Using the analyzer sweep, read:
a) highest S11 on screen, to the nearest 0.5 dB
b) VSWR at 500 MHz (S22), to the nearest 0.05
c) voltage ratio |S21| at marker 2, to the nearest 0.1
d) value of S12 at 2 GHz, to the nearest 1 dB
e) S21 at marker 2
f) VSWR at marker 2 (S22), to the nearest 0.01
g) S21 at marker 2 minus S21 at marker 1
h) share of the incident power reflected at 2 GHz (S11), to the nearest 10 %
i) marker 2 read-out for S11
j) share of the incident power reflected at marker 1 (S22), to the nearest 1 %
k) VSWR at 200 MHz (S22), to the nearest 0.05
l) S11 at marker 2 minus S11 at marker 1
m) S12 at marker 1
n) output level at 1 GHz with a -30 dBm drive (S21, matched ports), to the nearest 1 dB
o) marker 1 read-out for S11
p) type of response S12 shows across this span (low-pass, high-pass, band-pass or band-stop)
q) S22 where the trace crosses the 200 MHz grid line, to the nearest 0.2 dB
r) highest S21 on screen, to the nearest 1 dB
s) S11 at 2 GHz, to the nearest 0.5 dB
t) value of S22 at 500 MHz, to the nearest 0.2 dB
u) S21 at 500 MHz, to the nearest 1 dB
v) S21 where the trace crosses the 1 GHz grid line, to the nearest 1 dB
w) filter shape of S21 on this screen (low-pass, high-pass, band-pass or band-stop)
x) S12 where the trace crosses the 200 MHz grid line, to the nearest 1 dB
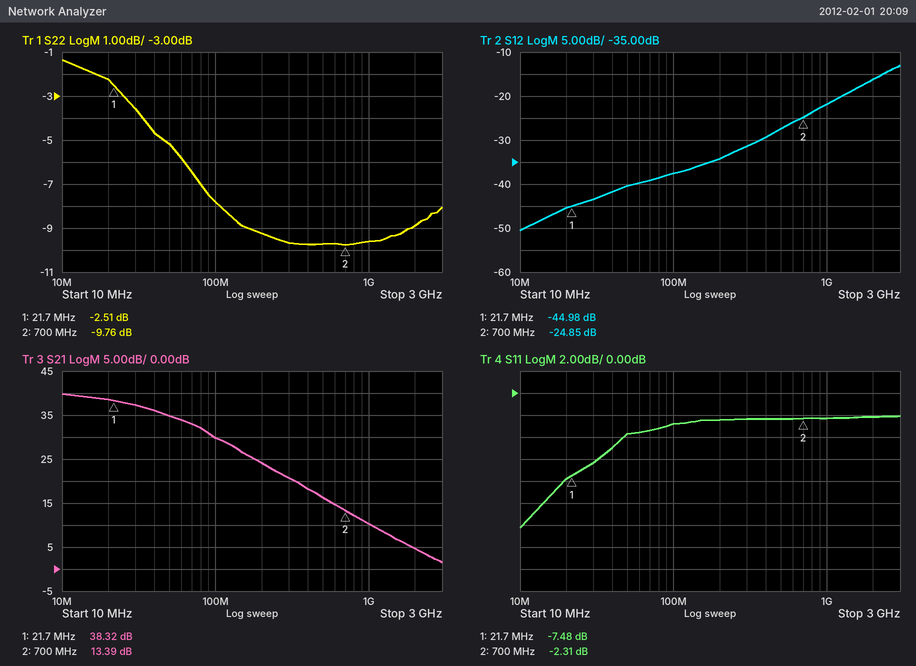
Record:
-2.0 dB
1.95
4.7
-16 dB
13.39 dB
1.96
-24.93 dB
60 %
-2.31 dB
56 %
2.05
5.17 dB
-44.98 dB
-20 dBm
-7.48 dB
high-pass
-9.2 dB
40 dB
-2.0 dB
-9.8 dB
16 dB
10 dB
low-pass
-34 dB
